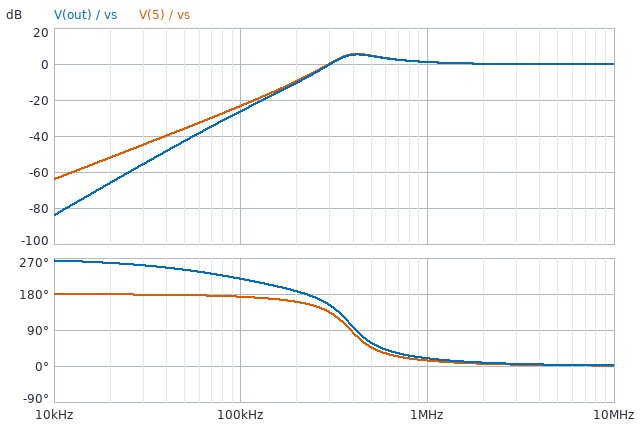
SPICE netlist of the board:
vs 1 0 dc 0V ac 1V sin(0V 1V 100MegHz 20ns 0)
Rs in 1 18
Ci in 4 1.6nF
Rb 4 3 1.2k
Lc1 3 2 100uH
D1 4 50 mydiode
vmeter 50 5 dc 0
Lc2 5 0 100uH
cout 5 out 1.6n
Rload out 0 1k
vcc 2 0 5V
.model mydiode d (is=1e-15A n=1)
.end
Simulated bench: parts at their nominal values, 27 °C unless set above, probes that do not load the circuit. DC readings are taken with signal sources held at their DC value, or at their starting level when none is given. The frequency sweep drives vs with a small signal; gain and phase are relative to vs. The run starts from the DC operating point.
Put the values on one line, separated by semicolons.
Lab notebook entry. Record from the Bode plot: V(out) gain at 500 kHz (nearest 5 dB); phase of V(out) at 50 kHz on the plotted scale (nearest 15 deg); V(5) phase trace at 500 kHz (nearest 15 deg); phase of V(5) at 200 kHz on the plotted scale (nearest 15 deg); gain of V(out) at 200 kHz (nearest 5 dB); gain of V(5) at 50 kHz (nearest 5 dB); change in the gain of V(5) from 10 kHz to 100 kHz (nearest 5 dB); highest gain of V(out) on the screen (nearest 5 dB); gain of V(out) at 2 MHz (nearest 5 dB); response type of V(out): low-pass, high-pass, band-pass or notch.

5 dB; 240 deg; 45 deg; 165 deg; -10 dB; -35 dB; 40 dB; 5 dB; 0 dB; high-pass
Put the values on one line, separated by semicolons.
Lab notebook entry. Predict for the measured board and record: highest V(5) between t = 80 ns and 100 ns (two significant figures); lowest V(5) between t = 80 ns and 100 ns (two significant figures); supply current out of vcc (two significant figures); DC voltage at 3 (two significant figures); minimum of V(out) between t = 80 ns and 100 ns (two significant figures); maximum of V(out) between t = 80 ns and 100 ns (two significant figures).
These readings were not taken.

970 mV; -980 mV; 3.5 mA; 5.0 V; -980 mV; 970 mV
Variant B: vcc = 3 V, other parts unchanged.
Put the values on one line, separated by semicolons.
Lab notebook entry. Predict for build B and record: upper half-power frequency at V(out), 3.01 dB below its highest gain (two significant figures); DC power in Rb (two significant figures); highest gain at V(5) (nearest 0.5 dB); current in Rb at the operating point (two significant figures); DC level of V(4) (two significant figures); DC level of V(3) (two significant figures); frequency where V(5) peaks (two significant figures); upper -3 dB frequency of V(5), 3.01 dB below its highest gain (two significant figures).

740 kHz; 4.3 mW; 5.0 dB; 1.9 mA; 730 mV; 3.0 V; 420 kHz; 720 kHz
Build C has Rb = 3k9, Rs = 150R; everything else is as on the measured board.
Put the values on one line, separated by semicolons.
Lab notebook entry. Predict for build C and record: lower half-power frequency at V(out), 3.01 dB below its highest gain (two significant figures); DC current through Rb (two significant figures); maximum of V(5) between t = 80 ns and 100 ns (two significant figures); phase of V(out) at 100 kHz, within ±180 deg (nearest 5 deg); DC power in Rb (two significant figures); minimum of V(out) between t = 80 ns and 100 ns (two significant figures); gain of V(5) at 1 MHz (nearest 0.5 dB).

300 kHz; 1.1 mA; 850 mV; -150 deg; 4.7 mW; -840 mV; -1.0 dB
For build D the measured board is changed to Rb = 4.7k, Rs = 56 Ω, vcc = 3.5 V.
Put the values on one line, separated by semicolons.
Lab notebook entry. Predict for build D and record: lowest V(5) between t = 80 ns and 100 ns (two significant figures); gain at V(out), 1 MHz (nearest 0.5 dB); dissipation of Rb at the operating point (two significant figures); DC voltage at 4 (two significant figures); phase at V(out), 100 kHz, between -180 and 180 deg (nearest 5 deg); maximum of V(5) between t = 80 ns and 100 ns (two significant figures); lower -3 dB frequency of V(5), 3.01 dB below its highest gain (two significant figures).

-650 mV; 0 dB; 1.7 mW; 700 mV; -145 deg; 920 mV; 310 kHz
